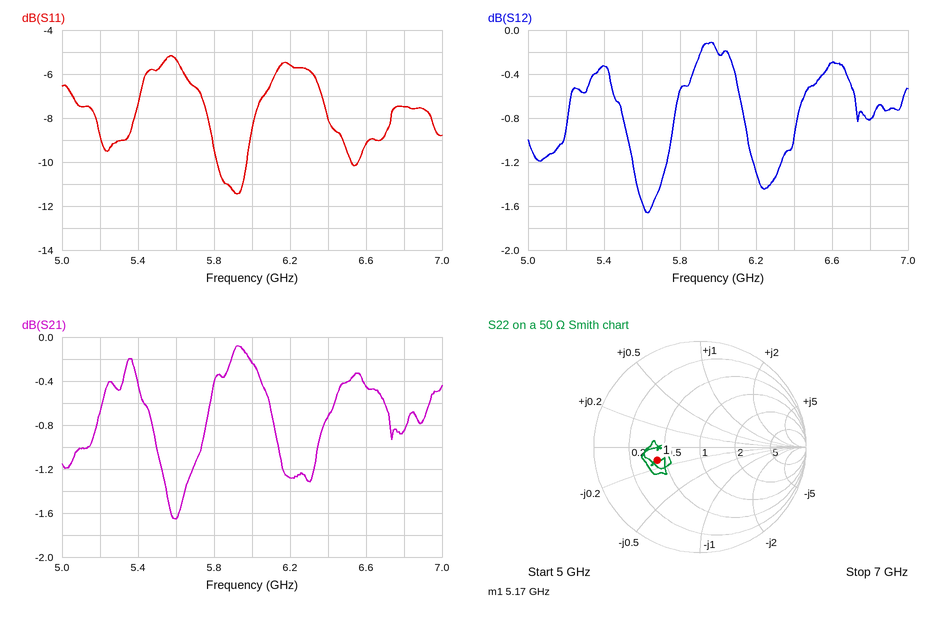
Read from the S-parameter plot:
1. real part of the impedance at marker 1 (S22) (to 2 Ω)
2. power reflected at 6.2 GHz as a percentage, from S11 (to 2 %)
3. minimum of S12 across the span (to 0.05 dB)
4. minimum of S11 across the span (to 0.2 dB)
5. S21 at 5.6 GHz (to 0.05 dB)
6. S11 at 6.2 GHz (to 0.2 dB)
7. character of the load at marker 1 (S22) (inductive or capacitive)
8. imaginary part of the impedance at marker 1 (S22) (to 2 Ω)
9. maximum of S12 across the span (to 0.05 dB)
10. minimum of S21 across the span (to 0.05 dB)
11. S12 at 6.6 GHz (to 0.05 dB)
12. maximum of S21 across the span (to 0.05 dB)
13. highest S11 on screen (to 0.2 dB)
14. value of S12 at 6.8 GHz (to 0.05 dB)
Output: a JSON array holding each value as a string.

["20 Ω", "28 %", "-1.65 dB", "-11.4 dB", "-1.65 dB", "-5.6 dB", "capacitive", "-6 Ω", "-0.10 dB", "-1.65 dB", "-0.30 dB", "-0.10 dB", "-5.2 dB", "-0.80 dB"]
